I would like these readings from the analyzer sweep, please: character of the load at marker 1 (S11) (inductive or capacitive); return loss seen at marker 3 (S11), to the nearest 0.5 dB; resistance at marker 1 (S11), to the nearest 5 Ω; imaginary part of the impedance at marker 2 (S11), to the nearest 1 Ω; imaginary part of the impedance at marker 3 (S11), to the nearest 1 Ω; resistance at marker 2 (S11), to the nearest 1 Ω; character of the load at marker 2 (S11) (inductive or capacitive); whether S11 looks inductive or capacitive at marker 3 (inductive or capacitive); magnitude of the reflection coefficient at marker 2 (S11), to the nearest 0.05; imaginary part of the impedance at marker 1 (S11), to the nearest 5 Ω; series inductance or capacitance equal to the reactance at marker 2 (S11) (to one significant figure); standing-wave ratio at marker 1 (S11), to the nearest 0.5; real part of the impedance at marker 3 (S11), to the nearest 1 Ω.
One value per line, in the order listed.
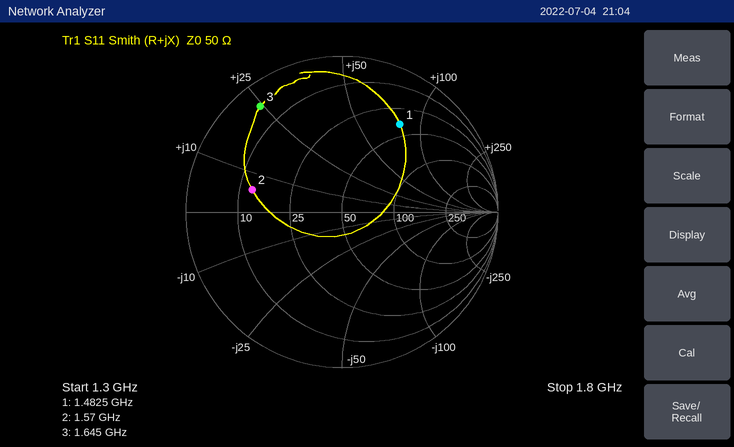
inductive
1.5 dB
40 Ω
+6 Ω
+24 Ω
13 Ω
inductive
inductive
0.60
+80 Ω
600 pH
5.0
5 Ω
